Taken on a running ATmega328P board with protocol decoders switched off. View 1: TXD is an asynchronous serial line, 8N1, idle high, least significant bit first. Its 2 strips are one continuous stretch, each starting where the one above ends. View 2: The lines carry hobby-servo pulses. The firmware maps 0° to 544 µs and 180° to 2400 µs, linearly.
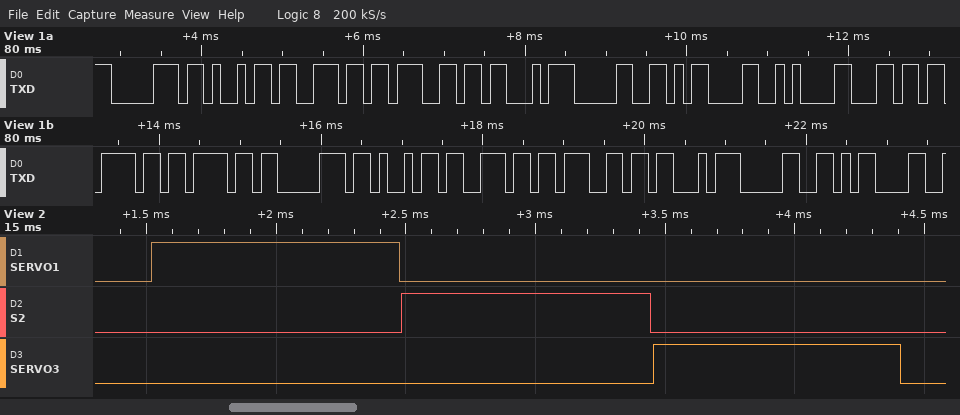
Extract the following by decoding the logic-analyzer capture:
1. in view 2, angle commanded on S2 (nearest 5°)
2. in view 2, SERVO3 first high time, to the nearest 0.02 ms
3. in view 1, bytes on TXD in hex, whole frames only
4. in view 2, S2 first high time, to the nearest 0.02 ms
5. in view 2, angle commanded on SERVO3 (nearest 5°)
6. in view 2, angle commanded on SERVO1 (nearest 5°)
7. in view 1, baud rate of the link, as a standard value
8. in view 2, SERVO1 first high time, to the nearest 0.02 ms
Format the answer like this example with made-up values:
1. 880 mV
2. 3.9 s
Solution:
1. 40°
2. 0.96 ms
3. 70 69 6E 67 A3 30 0D 0A 6C 6F 6F 70 69 6E 67 A3 30 0D
4. 0.96 ms
5. 40°
6. 40°
7. 9600 baud
8. 0.96 ms
